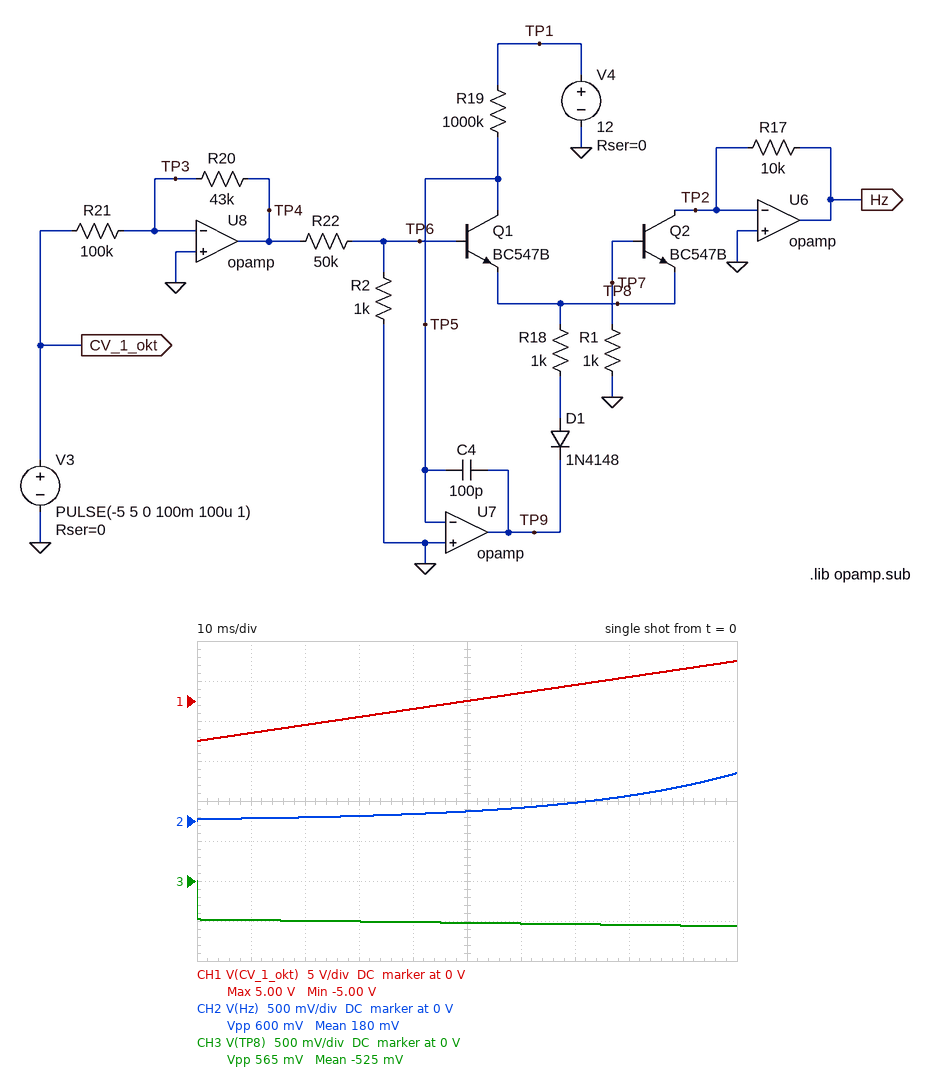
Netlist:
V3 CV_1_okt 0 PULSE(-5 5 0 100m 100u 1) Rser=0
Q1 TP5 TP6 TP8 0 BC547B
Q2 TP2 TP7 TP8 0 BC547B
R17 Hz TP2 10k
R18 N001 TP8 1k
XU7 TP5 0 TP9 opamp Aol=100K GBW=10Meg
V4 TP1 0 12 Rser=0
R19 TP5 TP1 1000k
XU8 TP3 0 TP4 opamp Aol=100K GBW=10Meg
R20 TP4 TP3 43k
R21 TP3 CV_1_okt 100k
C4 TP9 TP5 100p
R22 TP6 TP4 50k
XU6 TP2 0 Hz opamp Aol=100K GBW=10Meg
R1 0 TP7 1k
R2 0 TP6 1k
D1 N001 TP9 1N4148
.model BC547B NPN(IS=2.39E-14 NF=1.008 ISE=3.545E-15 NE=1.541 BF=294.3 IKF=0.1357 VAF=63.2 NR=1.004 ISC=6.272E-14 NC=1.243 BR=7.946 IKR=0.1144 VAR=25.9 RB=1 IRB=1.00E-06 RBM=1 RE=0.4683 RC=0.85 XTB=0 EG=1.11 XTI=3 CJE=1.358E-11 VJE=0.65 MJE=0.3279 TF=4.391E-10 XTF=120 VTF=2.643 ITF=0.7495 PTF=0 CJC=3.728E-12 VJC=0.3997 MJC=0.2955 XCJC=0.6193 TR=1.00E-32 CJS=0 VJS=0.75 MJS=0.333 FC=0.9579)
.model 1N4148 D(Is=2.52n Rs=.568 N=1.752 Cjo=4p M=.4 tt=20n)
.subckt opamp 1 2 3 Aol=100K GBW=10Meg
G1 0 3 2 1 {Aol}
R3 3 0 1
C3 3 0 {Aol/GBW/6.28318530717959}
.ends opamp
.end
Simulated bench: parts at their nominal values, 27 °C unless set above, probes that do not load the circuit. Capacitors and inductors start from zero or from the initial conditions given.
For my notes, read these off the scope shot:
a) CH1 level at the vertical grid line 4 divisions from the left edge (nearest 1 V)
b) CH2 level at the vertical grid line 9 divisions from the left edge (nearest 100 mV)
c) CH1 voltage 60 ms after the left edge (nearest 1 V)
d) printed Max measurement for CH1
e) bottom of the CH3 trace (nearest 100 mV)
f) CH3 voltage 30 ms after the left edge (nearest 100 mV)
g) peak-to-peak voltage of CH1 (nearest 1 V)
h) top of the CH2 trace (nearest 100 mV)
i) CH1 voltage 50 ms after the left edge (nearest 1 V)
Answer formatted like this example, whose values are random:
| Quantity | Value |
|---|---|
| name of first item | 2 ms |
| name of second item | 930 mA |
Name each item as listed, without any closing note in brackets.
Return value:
| Quantity | Value |
|---|---|
| CH1 level at the vertical grid line 4 divisions from the left edge | -1 V |
| CH2 level at the vertical grid line 9 divisions from the left edge | 400 mV |
| CH1 voltage 60 ms after the left edge | 1 V |
| printed Max measurement for CH1 | 5.00 V |
| bottom of the CH3 trace | -600 mV |
| CH3 voltage 30 ms after the left edge | -500 mV |
| peak-to-peak voltage of CH1 | 10 V |
| top of the CH2 trace | 600 mV |
| CH1 voltage 50 ms after the left edge | 0 V |
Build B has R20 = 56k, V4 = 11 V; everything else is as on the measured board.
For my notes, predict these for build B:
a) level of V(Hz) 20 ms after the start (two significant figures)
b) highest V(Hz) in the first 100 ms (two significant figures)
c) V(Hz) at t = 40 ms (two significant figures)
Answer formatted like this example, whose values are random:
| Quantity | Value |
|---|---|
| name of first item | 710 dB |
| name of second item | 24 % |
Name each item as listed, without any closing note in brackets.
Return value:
| Quantity | Value |
|---|---|
| level of V(Hz) 20 ms after the start | 31 mV |
| highest V(Hz) in the first 100 ms | 890 mV |
| V(Hz) at t = 40 ms | 72 mV |
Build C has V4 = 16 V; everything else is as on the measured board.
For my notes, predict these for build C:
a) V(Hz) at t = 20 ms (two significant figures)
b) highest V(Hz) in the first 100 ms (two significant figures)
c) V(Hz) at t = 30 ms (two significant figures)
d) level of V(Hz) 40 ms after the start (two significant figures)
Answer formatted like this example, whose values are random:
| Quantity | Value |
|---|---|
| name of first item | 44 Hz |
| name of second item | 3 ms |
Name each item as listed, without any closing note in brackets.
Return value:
| Quantity | Value |
|---|---|
| V(Hz) at t = 20 ms | 61 mV |
| highest V(Hz) in the first 100 ms | 800 mV |
| V(Hz) at t = 30 ms | 84 mV |
| level of V(Hz) 40 ms after the start | 120 mV |
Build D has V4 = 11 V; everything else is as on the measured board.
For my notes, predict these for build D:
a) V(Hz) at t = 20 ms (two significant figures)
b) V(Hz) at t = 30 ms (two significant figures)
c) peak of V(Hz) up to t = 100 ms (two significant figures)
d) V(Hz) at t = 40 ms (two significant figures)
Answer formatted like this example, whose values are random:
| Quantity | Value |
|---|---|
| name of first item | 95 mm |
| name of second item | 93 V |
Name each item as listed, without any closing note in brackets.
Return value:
| Quantity | Value |
|---|---|
| V(Hz) at t = 20 ms | 42 mV |
| V(Hz) at t = 30 ms | 58 mV |
| peak of V(Hz) up to t = 100 ms | 550 mV |
| V(Hz) at t = 40 ms | 80 mV |
